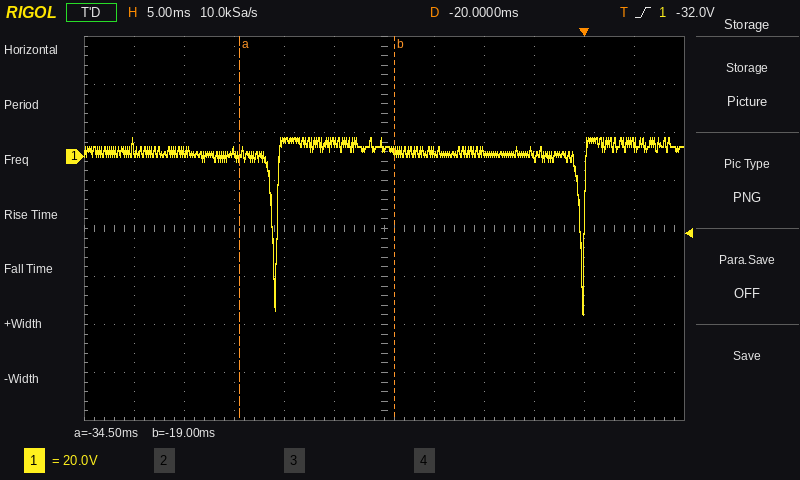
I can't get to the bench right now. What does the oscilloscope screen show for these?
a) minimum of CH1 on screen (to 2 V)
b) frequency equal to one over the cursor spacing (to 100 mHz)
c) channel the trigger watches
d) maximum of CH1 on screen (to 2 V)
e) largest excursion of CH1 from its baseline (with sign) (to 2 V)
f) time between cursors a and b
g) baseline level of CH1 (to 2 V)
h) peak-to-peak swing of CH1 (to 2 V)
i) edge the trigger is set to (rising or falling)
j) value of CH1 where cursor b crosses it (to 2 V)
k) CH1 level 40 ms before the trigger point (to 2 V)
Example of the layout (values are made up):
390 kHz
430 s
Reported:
-66 V
64.5 Hz
CH1
8 V
-68 V
15.5 ms
2 V
74 V
rising
2 V
2 V
